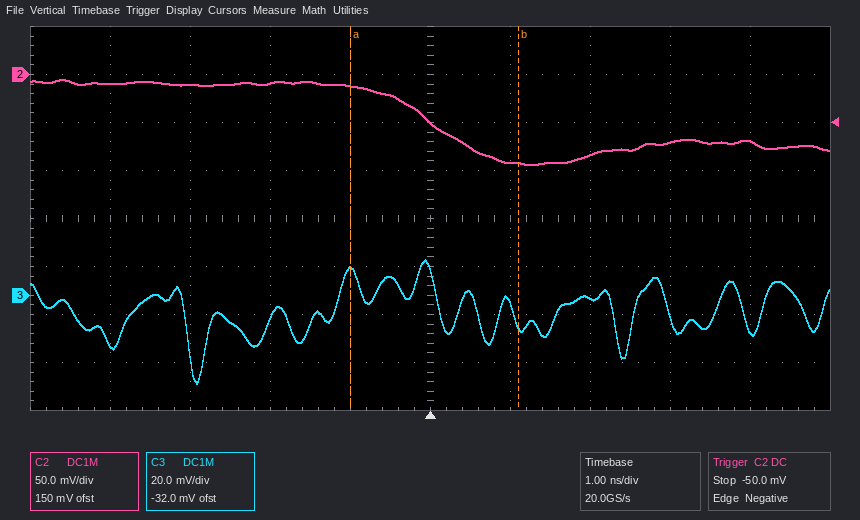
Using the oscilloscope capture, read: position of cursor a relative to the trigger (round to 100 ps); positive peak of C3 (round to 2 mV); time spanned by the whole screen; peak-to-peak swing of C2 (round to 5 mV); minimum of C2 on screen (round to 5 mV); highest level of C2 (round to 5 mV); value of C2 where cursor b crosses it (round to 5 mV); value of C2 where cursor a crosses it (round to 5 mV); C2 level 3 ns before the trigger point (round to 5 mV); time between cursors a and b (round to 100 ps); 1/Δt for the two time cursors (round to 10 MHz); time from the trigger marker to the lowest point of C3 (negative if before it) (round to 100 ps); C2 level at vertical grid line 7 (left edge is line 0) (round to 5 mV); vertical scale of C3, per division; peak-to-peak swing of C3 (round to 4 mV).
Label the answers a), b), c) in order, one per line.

a) -1.0 ns
b) 14 mV
c) 10 ns
d) 90 mV
e) -95 mV
f) -5 mV
g) -90 mV
h) -10 mV
i) -10 mV
j) 2.1 ns
k) 480 MHz
l) -2.9 ns
m) -85 mV
n) 20 mV
o) 52 mV
